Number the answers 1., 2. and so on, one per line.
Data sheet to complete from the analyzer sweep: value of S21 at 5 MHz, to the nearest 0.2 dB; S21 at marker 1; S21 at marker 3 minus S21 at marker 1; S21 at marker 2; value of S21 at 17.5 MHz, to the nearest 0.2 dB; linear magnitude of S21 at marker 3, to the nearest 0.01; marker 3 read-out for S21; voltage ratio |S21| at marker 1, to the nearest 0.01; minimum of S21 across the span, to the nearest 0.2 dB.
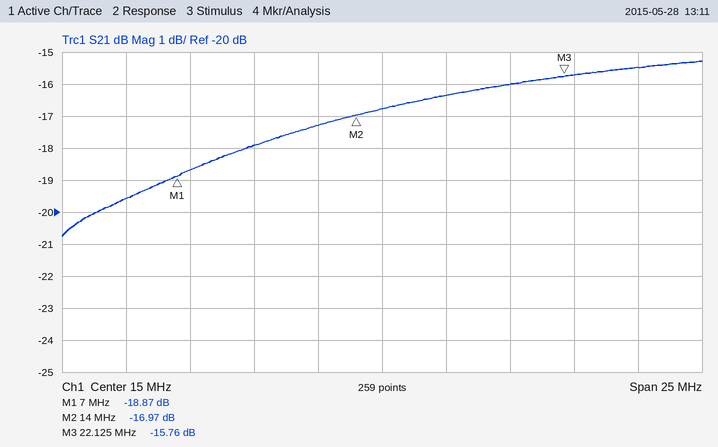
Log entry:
1. -19.6 dB
2. -18.87 dB
3. 3.11 dB
4. -16.97 dB
5. -16.4 dB
6. 0.16
7. -15.76 dB
8. 0.11
9. -20.8 dB
